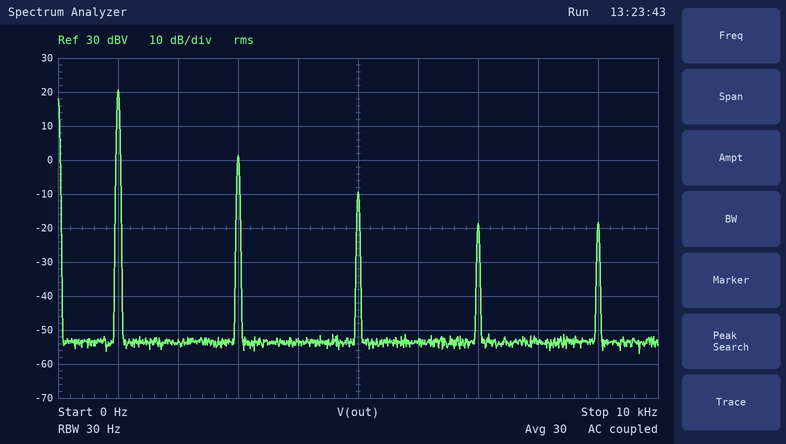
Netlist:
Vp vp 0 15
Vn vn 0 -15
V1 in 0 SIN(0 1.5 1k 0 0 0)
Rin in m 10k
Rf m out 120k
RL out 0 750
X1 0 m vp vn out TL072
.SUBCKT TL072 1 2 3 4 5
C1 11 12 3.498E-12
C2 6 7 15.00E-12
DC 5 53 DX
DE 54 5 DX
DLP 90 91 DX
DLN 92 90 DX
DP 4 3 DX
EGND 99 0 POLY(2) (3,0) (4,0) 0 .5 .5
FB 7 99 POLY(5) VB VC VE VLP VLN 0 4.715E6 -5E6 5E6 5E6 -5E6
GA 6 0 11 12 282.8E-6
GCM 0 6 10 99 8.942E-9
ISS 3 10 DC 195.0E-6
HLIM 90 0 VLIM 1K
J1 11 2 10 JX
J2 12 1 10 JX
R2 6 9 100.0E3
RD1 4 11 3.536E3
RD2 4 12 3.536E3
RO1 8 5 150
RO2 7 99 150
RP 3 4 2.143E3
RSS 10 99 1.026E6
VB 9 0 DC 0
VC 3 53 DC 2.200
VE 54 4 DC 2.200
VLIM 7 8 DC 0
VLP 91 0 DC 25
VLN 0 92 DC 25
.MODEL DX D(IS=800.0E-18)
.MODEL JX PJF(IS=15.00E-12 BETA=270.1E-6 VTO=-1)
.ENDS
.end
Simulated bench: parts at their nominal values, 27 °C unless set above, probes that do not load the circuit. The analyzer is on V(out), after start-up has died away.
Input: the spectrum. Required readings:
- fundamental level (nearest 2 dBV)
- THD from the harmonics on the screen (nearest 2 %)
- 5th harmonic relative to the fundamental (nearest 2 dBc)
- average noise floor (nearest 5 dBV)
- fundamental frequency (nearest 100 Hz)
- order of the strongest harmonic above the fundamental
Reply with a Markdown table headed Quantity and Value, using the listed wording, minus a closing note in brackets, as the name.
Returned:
| Quantity | Value |
|---|---|
| fundamental level | 20 dBV |
| THD from the harmonics on the screen | 12 % |
| 5th harmonic relative to the fundamental | -30 dBc |
| average noise floor | -55 dBV |
| fundamental frequency | 1.0 kHz |
| order of the strongest harmonic above the fundamental | 3 |
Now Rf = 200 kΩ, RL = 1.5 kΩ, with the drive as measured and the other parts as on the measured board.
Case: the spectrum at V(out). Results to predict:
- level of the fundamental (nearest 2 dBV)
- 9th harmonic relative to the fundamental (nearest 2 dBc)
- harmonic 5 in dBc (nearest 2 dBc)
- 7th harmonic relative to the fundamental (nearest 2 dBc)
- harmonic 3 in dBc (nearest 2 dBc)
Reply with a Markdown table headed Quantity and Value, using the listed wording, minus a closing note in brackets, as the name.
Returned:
| Quantity | Value |
|---|---|
| level of the fundamental | 22 dBV |
| 9th harmonic relative to the fundamental | -34 dBc |
| harmonic 5 in dBc | -24 dBc |
| 7th harmonic relative to the fundamental | -56 dBc |
| harmonic 3 in dBc | -12 dBc |
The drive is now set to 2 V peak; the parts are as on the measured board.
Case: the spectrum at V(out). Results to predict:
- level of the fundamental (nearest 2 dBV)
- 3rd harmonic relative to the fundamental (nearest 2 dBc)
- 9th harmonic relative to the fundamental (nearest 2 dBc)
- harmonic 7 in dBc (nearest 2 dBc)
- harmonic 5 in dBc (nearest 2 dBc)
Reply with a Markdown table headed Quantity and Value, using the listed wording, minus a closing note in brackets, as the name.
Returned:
| Quantity | Value |
|---|---|
| level of the fundamental | 22 dBV |
| 3rd harmonic relative to the fundamental | -14 dBc |
| 9th harmonic relative to the fundamental | -36 dBc |
| harmonic 7 in dBc | -32 dBc |
| harmonic 5 in dBc | -34 dBc |
